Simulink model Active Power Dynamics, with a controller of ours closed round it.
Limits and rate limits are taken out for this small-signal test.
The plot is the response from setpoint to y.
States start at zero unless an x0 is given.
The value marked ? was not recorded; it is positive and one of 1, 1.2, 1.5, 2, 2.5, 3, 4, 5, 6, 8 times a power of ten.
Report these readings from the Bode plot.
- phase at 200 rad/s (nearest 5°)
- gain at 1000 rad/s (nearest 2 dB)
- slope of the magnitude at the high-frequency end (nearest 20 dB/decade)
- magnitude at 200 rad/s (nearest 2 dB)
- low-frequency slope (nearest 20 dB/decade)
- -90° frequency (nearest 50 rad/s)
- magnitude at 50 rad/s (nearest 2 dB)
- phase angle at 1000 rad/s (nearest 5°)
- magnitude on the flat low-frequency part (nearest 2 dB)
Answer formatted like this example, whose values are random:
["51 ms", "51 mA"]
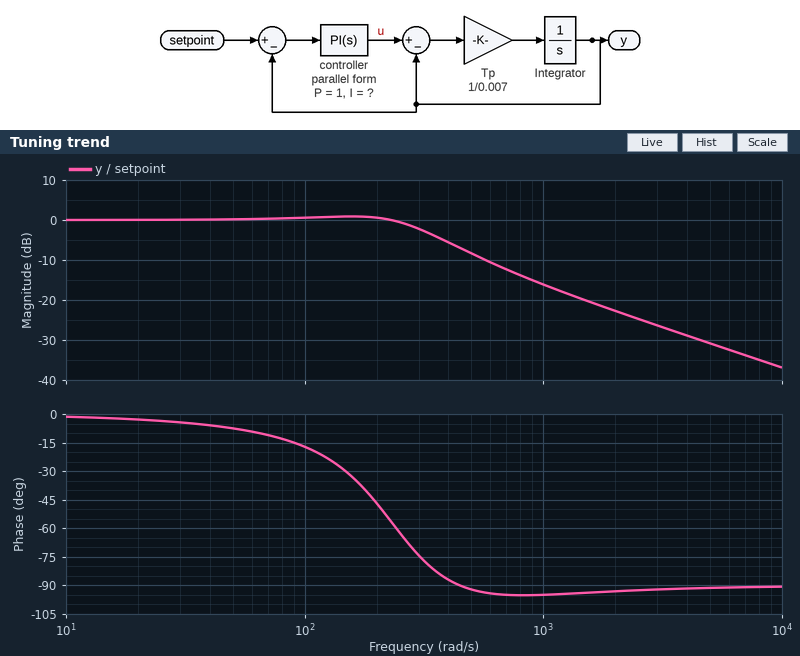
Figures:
["-45°", "-16 dB", "-20 dB/decade", "0 dB", "0 dB/decade", "450 rad/s", "0 dB", "-95°", "0 dB"]
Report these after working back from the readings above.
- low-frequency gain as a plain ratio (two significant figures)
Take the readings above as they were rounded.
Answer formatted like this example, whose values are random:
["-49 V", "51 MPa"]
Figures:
["1.0"]
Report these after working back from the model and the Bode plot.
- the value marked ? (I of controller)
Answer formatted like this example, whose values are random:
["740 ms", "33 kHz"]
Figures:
["400"]
